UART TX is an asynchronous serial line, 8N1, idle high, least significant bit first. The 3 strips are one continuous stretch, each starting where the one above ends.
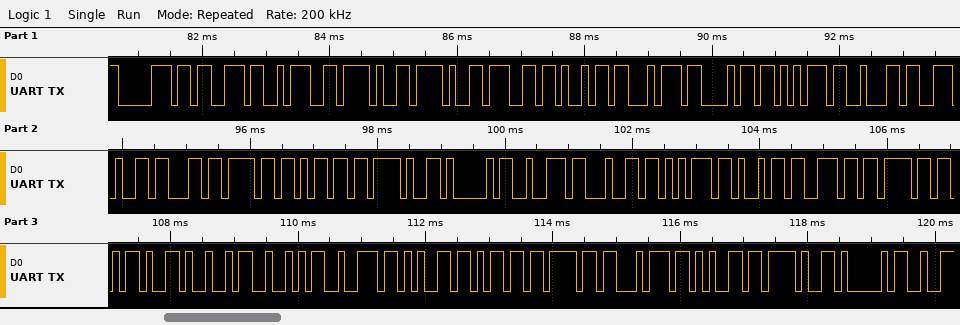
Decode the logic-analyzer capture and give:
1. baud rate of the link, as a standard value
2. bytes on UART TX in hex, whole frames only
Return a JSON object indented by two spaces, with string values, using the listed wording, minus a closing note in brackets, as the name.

{
  "baud rate of the link, as a standard value": "9600 baud",
  "bytes on UART TX in hex, whole frames only": "70 73 3A 2F 2F 67 69 74 68 75 62 2E 63 6F 6D 2F 41 72 64 75 69 6E 6F 2D 49 52 72 65 6D 6F 74 65 2F 41"
}
